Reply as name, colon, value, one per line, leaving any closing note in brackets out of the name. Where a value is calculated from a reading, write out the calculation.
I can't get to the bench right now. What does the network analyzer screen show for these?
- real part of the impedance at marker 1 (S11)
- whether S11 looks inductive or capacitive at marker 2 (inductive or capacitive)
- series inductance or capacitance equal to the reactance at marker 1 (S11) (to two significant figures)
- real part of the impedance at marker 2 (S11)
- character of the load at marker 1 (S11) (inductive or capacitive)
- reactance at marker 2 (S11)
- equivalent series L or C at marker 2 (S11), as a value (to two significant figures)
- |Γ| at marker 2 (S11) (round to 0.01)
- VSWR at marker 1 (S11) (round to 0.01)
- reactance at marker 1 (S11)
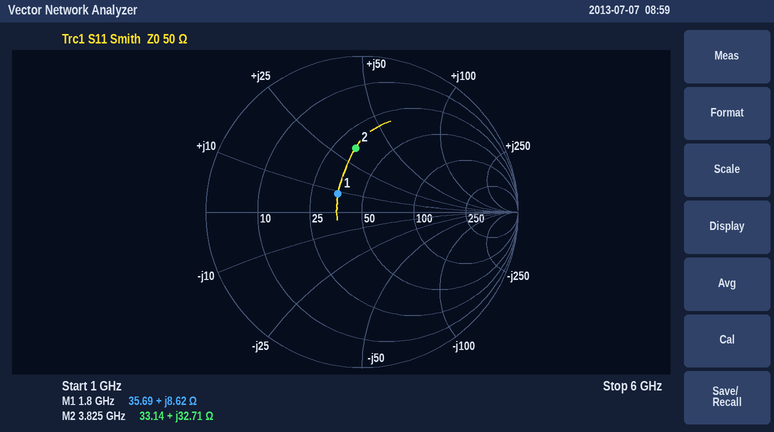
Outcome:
real part of the impedance at marker 1: 35.69 Ω
whether S11 looks inductive or capacitive at marker 2: inductive
series inductance or capacitance equal to the reactance at marker 1 (S11): L = 8.62 Ω/(2π × 1.8 GHz) ≈ 762 pH, so 760 pH to two significant figures
real part of the impedance at marker 2: 33.14 Ω
character of the load at marker 1 (S11): inductive
reactance at marker 2: +32.71 Ω
equivalent series L or C at marker 2 (S11), as a value: L = 32.71 Ω/(2π × 3.825 GHz) ≈ 1.4 nH
|Γ| at marker 2 (S11): 0.41
VSWR at marker 1 (S11): 1.48
reactance at marker 1: +8.62 Ω
